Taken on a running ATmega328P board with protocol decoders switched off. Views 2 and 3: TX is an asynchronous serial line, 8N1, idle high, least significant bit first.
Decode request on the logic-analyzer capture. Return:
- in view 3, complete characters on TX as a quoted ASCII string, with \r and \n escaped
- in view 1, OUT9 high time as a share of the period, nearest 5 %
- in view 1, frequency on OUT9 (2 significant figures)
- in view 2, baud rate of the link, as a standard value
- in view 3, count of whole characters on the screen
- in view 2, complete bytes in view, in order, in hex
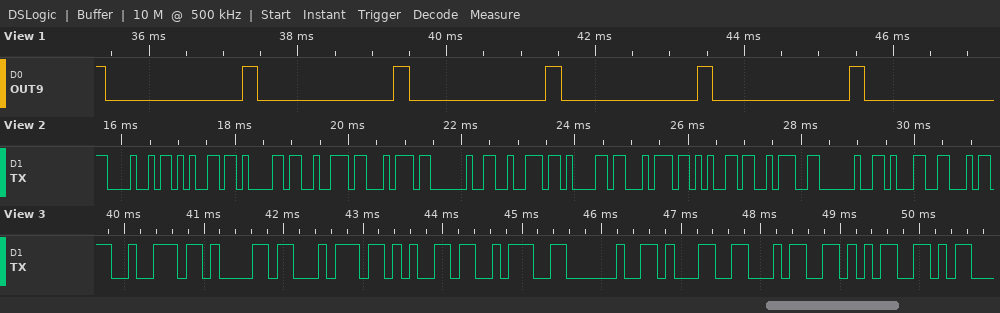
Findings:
"rate: 145"
10 %
490 Hz
9600 baud
9
48 65 61 72 74 20 72 61 74 65 3A 20 31
